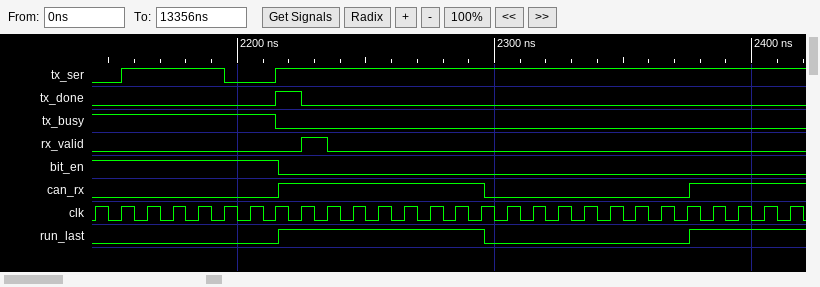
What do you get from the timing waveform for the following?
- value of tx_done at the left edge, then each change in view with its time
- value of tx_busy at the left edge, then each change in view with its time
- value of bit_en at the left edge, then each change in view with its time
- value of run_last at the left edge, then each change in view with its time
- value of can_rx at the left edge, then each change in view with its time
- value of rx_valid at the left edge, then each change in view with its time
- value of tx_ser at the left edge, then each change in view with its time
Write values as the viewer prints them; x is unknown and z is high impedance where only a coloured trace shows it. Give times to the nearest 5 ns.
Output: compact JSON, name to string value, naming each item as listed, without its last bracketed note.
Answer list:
{"value of tx_done at the left edge, then each change in view with its time": "0, 1 at 2215 ns, 0 at 2225 ns", "value of tx_busy at the left edge, then each change in view with its time": "1, 0 at 2215 ns", "value of bit_en at the left edge, then each change in view with its time": "1, 0 at 2215 ns", "value of run_last at the left edge, then each change in view with its time": "0, 1 at 2215 ns, 0 at 2295 ns, 1 at 2375 ns", "value of can_rx at the left edge, then each change in view with its time": "0, 1 at 2215 ns, 0 at 2295 ns, 1 at 2375 ns", "value of rx_valid at the left edge, then each change in view with its time": "0, 1 at 2225 ns, 0 at 2235 ns", "value of tx_ser at the left edge, then each change in view with its time": "0, 1 at 2155 ns, 0 at 2195 ns, 1 at 2215 ns"}
